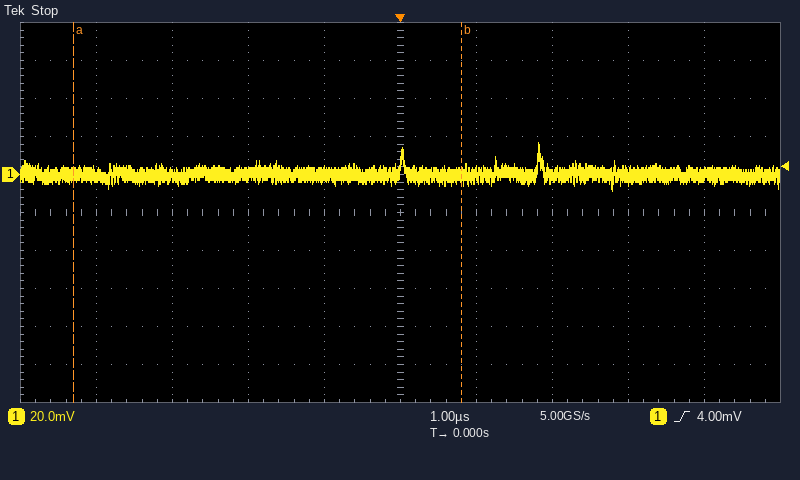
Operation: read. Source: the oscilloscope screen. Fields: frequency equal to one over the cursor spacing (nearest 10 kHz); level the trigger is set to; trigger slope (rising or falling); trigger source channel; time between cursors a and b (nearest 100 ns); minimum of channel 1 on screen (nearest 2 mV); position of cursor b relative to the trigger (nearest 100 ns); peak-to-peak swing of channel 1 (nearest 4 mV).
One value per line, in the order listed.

200 kHz
4.00 mV
rising
channel 1
5.1 µs
-8 mV
+800 ns
24 mV
